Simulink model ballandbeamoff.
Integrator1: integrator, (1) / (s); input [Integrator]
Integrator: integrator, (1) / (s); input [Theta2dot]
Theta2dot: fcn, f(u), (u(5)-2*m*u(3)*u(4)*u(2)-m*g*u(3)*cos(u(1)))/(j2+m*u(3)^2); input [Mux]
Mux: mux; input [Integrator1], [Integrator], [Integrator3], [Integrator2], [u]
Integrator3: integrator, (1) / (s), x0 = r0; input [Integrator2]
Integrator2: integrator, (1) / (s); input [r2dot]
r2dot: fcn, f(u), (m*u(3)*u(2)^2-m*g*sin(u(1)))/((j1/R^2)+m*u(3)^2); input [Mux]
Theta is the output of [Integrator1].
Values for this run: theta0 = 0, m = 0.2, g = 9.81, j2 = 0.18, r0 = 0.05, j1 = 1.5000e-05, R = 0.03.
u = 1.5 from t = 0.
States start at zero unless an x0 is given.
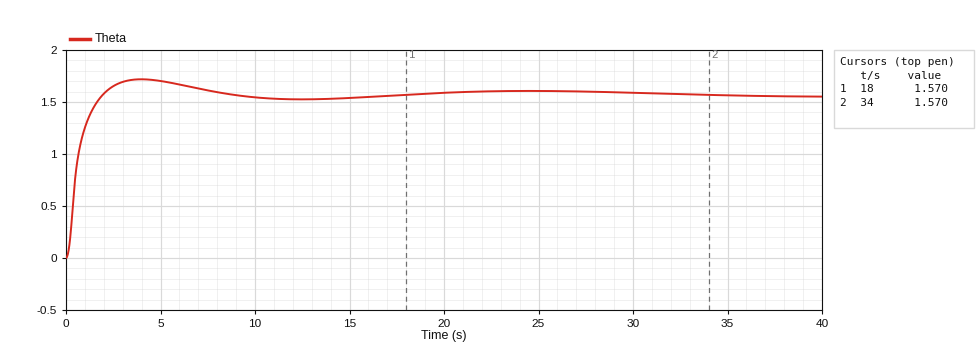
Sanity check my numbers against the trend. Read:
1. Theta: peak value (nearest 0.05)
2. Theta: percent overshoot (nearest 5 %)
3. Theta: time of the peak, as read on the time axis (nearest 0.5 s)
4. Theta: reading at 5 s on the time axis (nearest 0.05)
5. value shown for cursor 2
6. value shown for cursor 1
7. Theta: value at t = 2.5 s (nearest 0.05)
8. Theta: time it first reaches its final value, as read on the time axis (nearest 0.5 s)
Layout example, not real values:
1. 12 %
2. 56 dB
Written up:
1. 1.70
2. 10 %
3. 4.0 s
4. 1.70
5. 1.570
6. 1.570
7. 1.65
8. 2.0 s
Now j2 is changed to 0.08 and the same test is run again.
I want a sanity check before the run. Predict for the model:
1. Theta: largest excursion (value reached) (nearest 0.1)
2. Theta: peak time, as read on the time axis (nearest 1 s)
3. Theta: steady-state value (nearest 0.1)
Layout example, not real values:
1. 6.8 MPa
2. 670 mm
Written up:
1. 1.7
2. 5 s
3. 1.6
